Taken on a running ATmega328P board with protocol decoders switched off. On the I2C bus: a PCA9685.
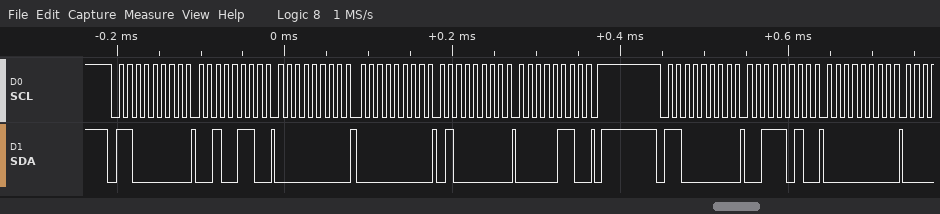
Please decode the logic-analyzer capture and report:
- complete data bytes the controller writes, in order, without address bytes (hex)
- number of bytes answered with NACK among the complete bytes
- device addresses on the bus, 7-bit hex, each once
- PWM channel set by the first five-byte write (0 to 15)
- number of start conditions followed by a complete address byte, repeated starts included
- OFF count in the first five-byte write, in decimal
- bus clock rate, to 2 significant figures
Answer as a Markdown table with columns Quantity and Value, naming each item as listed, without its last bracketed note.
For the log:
| Quantity | Value |
|---|---|
| complete data bytes the controller writes, in order, without address bytes | 26 00 00 40 06 3A 00 |
| number of bytes answered with NACK among the complete bytes | 0 |
| device addresses on the bus, 7-bit hex, each once | 0x60 |
| PWM channel set by the first five-byte write | 8 |
| number of start conditions followed by a complete address byte, repeated starts included | 2 |
| OFF count in the first five-byte write, in decimal | 1600 |
| bus clock rate, to 2 significant figures | 100 kHz |
